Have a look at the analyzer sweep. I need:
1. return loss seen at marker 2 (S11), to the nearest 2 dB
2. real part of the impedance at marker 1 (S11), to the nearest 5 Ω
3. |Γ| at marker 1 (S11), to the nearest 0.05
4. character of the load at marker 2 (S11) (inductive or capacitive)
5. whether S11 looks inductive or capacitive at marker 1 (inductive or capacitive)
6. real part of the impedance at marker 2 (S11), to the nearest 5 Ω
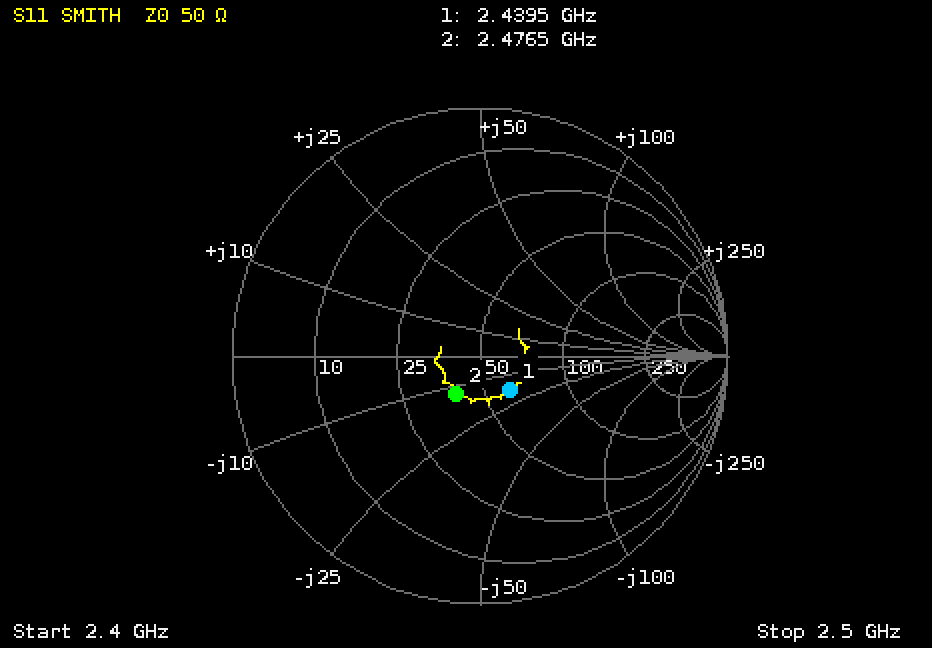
14 dB
60 Ω
0.20
capacitive
capacitive
40 Ω
